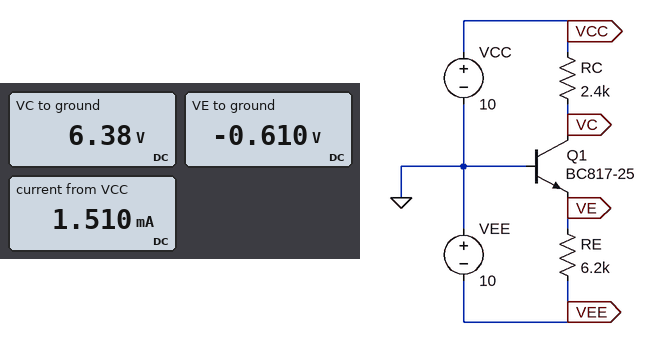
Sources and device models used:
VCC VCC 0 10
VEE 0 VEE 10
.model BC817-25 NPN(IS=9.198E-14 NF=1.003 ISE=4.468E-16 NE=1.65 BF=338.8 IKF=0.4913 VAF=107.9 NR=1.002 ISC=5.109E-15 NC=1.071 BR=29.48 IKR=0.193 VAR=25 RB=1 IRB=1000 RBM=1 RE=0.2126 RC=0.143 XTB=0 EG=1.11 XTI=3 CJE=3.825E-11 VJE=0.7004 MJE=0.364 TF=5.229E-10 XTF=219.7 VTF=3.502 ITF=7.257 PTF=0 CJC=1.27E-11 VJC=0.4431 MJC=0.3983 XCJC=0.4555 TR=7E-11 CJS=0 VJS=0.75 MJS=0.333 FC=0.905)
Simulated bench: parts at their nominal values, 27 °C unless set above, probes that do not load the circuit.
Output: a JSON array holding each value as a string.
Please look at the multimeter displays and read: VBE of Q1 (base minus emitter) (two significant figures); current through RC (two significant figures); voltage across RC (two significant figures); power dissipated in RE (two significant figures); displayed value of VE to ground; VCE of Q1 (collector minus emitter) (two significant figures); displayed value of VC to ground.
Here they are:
["610 mV", "1.5 mA", "3.6 V", "14 mW", "-0.610 V", "7.0 V", "6.38 V"]
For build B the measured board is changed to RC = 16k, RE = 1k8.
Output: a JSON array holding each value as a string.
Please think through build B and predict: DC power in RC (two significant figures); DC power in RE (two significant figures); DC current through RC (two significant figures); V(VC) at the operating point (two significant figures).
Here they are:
["7.2 mW", "48 mW", "670 µA", "-720 mV"]
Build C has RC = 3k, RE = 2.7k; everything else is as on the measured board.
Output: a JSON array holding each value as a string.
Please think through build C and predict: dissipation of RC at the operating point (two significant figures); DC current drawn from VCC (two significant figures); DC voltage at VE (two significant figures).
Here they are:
["36 mW", "3.5 mA", "-630 mV"]
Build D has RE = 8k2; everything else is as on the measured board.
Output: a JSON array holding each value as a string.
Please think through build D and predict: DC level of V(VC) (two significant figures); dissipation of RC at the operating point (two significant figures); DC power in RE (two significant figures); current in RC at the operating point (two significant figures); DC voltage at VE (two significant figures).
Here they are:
["7.3 V", "3.1 mW", "11 mW", "1.1 mA", "-600 mV"]
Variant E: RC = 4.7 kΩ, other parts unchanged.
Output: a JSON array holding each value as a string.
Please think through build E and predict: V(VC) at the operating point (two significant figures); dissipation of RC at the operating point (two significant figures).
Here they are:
["2.9 V", "11 mW"]
